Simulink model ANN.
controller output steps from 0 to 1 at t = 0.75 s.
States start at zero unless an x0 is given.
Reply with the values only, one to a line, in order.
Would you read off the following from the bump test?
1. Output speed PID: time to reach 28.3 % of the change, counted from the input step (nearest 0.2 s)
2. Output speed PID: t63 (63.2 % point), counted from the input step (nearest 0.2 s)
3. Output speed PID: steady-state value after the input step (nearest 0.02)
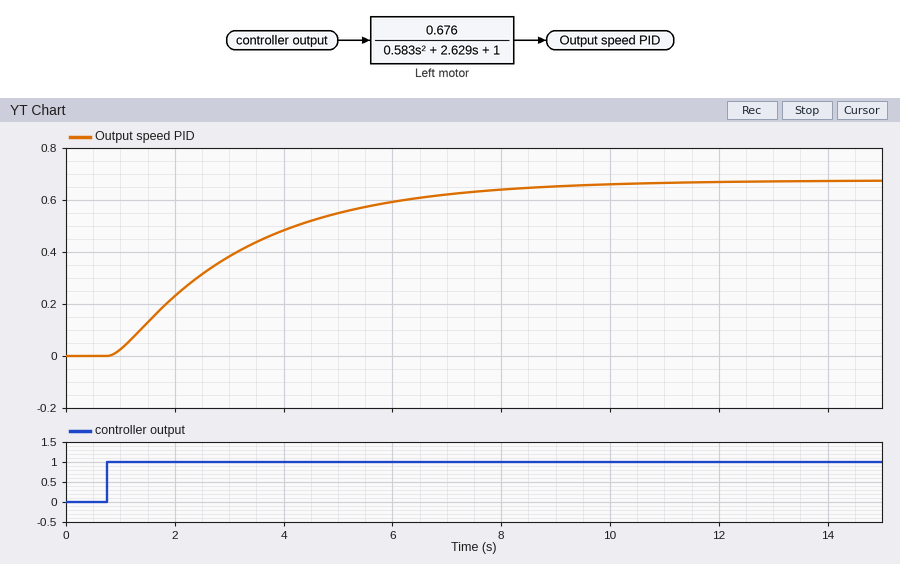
1.0 s
2.6 s
0.68
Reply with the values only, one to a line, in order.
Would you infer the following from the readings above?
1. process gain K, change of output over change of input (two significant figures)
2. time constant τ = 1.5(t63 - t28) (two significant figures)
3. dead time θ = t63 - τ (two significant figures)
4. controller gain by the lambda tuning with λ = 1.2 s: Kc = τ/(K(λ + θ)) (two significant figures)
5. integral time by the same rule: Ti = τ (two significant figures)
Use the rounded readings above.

0.68
2.4 s
0.20 s
2.5
2.4 s
